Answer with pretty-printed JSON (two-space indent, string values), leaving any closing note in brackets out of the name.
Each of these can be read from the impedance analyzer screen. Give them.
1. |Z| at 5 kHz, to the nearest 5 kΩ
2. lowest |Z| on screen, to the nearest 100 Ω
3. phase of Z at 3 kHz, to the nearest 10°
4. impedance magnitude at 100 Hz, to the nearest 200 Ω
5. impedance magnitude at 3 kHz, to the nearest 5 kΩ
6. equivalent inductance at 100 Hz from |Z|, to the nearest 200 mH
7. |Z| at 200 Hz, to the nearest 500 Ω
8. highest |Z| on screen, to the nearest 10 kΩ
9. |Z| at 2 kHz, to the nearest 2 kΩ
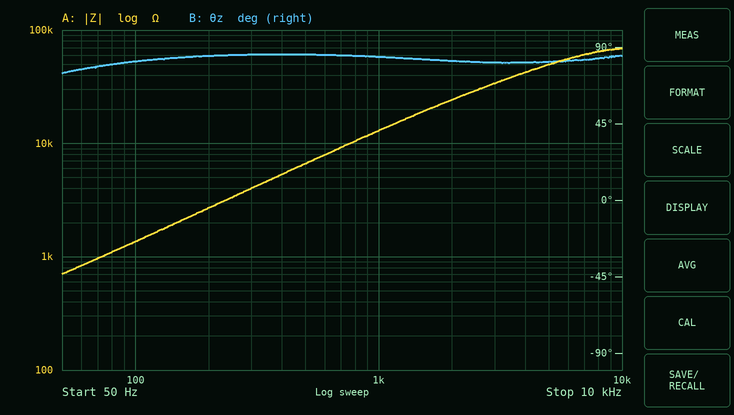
{
  "|Z| at 5 kHz, to the nearest 5 kΩ": "50 kΩ",
  "lowest |Z| on screen, to the nearest 100 Ω": "700 Ω",
  "phase of Z at 3 kHz, to the nearest 10°": "80°",
  "impedance magnitude at 100 Hz, to the nearest 200 Ω": "1.4 kΩ",
  "impedance magnitude at 3 kHz, to the nearest 5 kΩ": "35 kΩ",
  "equivalent inductance at 100 Hz from |Z|, to the nearest 200 mH": "2.2 H",
  "|Z| at 200 Hz, to the nearest 500 Ω": "2.5 kΩ",
  "highest |Z| on screen, to the nearest 10 kΩ": "70 kΩ",
  "|Z| at 2 kHz, to the nearest 2 kΩ": "24 kΩ"
}
